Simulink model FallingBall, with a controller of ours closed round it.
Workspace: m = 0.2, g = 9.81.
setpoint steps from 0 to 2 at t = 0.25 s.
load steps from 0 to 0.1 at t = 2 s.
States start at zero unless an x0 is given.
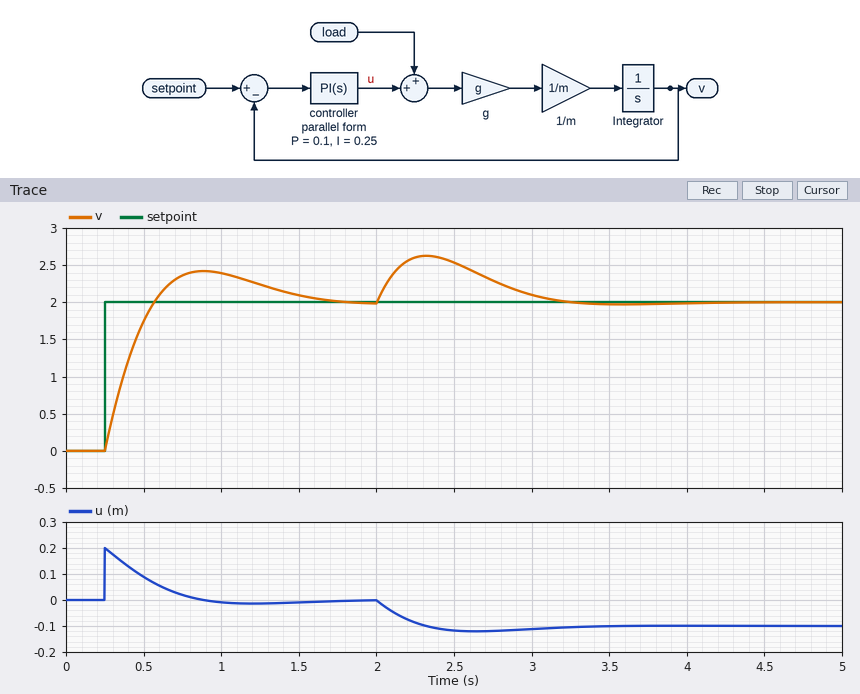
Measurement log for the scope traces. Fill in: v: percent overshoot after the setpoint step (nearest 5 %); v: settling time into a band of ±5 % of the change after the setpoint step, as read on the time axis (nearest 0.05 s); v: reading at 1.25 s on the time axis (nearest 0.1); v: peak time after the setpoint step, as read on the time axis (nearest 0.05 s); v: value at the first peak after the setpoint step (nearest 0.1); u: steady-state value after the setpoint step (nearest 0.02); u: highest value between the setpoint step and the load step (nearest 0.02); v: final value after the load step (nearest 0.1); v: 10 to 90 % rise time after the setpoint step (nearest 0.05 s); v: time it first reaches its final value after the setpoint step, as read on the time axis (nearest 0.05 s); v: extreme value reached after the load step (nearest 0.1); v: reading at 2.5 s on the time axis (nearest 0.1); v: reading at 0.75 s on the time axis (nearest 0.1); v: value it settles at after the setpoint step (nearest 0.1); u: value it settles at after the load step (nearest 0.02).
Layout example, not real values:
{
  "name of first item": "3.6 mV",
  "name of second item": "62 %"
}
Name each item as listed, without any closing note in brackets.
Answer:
{
  "v: percent overshoot after the setpoint step": "20 %",
  "v: settling time into a band of ±5 % of the change after the setpoint step, as read on the time axis": "1.50 s",
  "v: reading at 1.25 s on the time axis": "2.2",
  "v: peak time after the setpoint step, as read on the time axis": "0.90 s",
  "v: value at the first peak after the setpoint step": "2.4",
  "u: steady-state value after the setpoint step": "0.00",
  "u: highest value between the setpoint step and the load step": "0.20",
  "v: final value after the load step": "2.0",
  "v: 10 to 90 % rise time after the setpoint step": "0.25 s",
  "v: time it first reaches its final value after the setpoint step, as read on the time axis": "0.55 s",
  "v: extreme value reached after the load step": "2.6",
  "v: reading at 2.5 s on the time axis": "2.5",
  "v: reading at 0.75 s on the time axis": "2.4",
  "v: value it settles at after the setpoint step": "2.0",
  "u: value it settles at after the load step": "-0.10"
}
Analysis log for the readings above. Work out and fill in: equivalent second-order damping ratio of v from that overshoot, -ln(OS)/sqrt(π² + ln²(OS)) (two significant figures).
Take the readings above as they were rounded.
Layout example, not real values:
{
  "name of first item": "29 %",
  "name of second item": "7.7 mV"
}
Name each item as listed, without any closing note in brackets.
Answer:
{
  "equivalent second-order damping ratio of v from that overshoot, -ln(OS)/sqrt(π² + ln²(OS))": "0.46"
}
